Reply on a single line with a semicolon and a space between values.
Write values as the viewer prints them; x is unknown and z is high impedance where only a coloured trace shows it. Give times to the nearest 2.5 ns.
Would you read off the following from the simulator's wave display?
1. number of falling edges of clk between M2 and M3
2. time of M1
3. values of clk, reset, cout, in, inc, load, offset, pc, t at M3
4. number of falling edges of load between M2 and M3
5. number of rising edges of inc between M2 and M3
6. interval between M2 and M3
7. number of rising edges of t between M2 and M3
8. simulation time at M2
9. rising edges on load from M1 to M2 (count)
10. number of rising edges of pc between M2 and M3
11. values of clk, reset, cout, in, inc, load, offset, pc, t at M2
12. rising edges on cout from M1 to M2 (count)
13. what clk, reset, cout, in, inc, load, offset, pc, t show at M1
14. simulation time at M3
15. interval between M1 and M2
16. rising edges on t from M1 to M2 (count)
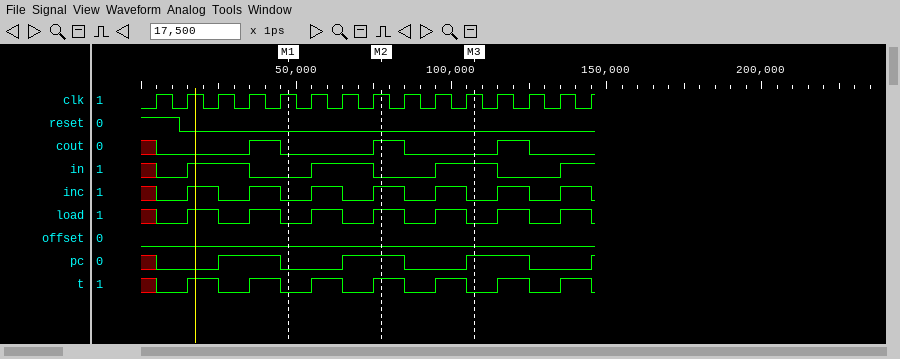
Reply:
3; 47.5 ns; clk=1, reset=0, cout=0, in=1, inc=0, load=0, offset=0, pc=1, t=0; 2; 1; 30 ns; 1; 77.5 ns; 2; 1; clk=1, reset=0, cout=1, in=0, inc=1, load=1, offset=0, pc=1, t=1; 1; clk=1, reset=0, cout=0, in=0, inc=0, load=0, offset=0, pc=0, t=0; 107.5 ns; 30 ns; 2
